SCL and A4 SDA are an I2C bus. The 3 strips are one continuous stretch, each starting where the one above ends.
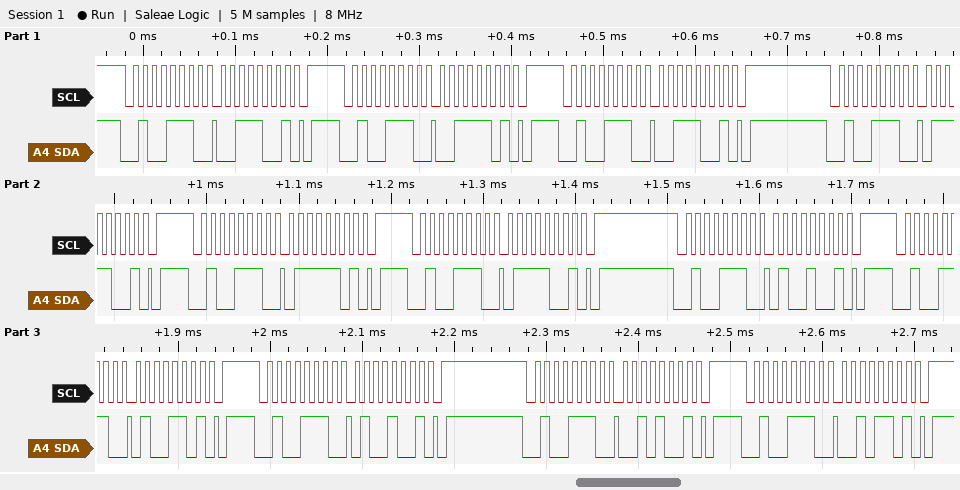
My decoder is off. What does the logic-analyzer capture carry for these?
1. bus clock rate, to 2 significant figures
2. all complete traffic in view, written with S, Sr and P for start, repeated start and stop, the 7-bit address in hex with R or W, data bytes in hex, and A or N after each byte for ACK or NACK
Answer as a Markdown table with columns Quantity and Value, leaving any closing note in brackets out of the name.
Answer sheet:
| Quantity | Value |
|---|---|
| bus clock rate, to 2 significant figures | 100 kHz |
| all complete traffic in view, written with S, Sr and P for start, repeated start and stop, the 7-bit address in hex with R or W, data bytes in hex, and A or N after each byte for ACK or NACK | S 27W A 39 A P S 27W A 3D A P S 27W A 39 A P S 27W A 79 A P S 27W A 7D A P S 27W A 79 A P S 27W A 49 A P S 27W A 4D A P S 27W A 49 A P S 27W A 29 A P S 27W A 2D A P |
